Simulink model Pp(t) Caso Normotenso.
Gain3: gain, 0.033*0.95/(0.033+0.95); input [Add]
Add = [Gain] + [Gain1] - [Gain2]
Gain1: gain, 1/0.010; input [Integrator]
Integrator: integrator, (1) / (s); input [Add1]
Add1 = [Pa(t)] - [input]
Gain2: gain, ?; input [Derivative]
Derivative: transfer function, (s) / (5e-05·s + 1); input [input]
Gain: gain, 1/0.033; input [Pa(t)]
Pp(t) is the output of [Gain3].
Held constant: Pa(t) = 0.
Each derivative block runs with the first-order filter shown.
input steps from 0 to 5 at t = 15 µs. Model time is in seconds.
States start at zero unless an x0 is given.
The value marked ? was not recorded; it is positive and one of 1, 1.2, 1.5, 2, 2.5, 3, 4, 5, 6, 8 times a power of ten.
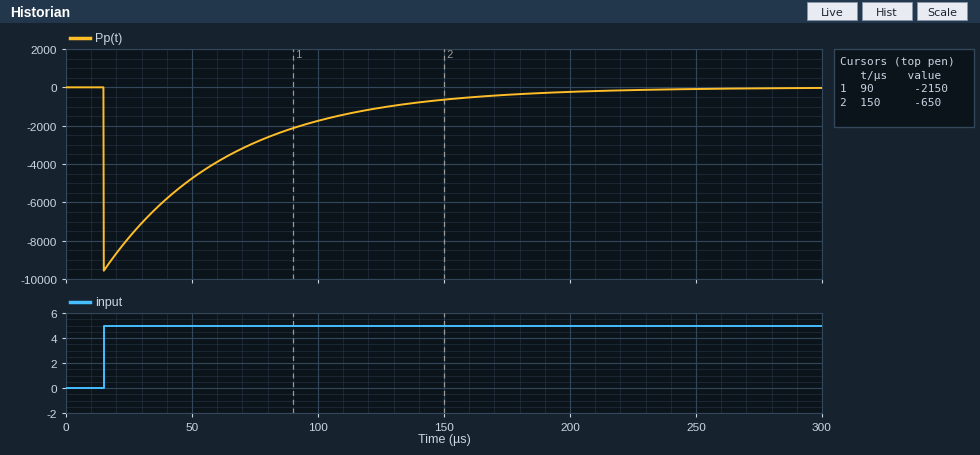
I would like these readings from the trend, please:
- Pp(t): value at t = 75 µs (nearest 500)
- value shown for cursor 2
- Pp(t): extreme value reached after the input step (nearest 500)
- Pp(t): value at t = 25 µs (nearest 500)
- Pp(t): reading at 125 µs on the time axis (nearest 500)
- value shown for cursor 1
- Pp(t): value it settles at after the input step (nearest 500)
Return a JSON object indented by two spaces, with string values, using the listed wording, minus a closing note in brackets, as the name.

{
  "Pp(t): value at t = 75 µs": "-3000",
  "value shown for cursor 2": "-650",
  "Pp(t): extreme value reached after the input step": "-9500",
  "Pp(t): value at t = 25 µs": "-8000",
  "Pp(t): reading at 125 µs on the time axis": "-1000",
  "value shown for cursor 1": "-2150",
  "Pp(t): value it settles at after the input step": "0"
}
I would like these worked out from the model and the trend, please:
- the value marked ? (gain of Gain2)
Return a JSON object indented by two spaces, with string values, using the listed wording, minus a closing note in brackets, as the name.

{
  "the value marked ?": "3"
}
